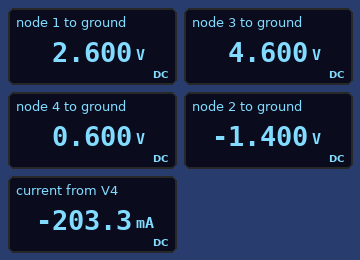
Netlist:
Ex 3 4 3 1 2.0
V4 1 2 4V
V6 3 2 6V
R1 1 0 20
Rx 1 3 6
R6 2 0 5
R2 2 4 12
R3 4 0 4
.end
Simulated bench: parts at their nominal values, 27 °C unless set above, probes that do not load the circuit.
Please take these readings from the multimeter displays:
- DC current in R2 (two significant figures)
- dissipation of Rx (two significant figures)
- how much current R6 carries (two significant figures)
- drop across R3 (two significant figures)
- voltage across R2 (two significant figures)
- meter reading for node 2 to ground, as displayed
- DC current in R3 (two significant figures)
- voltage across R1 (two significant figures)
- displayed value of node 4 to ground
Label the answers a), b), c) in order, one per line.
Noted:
a) 170 mA
b) 670 mW
c) 280 mA
d) 600 mV
e) 2.0 V
f) -1.400 V
g) 150 mA
h) 2.6 V
i) 0.600 V
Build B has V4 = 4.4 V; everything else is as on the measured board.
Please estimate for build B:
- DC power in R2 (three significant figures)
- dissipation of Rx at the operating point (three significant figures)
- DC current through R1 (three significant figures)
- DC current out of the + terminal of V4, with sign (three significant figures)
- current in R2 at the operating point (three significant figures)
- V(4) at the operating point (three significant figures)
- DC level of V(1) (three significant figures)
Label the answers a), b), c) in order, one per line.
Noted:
a) 653 mW
b) 427 mW
c) 128 mA
d) -139 mA
e) 233 mA
f) 960 mV
g) 2.56 V
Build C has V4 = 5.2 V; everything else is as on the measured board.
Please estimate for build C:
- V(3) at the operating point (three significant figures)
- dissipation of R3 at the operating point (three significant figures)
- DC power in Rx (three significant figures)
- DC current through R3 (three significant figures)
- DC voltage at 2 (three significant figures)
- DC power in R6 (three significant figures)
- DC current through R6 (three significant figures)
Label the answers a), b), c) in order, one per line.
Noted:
a) 3.28 V
b) 706 mW
c) 107 mW
d) 420 mA
e) -2.72 V
f) 1.48 W
g) 544 mA
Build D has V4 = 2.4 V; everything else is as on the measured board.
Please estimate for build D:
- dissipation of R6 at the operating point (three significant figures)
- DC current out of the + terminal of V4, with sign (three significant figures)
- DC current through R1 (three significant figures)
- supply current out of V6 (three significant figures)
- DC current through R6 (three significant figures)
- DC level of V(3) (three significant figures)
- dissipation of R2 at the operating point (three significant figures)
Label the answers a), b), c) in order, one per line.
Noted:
a) 25.9 mW
b) -462 mA
c) 138 mA
d) 290 mA
e) 72.0 mA
f) 6.36 V
g) 120 mW
